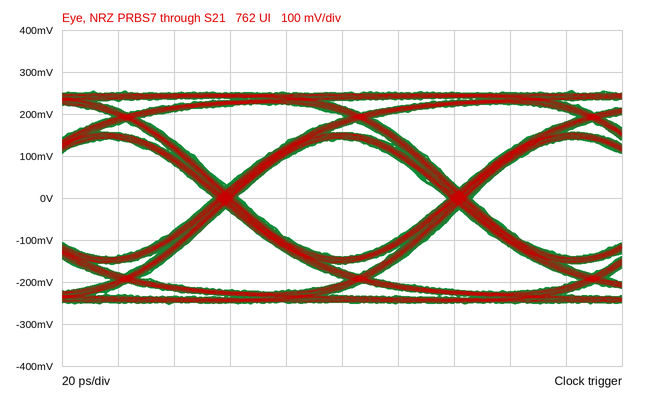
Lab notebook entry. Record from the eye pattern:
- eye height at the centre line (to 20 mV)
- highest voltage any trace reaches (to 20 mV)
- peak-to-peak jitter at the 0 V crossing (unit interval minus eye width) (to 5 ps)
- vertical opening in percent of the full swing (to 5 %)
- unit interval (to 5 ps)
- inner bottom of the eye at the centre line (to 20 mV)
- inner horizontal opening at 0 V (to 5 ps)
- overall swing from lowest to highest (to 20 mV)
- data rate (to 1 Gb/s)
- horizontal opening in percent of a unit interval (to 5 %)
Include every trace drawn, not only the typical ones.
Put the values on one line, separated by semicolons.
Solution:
280 mV; 260 mV; 10 ps; 55 %; 85 ps; -140 mV; 75 ps; 500 mV; 12 Gb/s; 90 %
